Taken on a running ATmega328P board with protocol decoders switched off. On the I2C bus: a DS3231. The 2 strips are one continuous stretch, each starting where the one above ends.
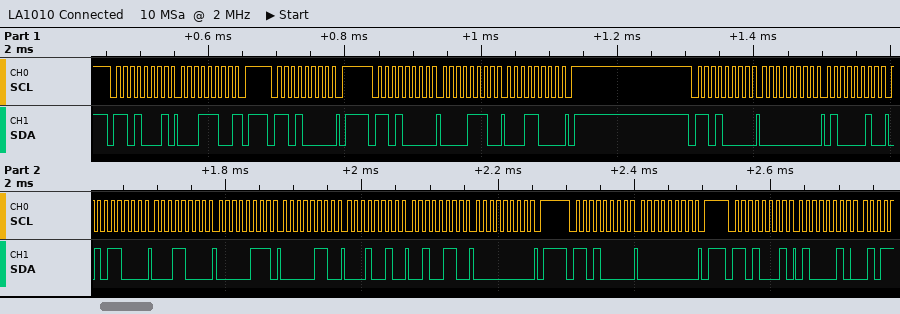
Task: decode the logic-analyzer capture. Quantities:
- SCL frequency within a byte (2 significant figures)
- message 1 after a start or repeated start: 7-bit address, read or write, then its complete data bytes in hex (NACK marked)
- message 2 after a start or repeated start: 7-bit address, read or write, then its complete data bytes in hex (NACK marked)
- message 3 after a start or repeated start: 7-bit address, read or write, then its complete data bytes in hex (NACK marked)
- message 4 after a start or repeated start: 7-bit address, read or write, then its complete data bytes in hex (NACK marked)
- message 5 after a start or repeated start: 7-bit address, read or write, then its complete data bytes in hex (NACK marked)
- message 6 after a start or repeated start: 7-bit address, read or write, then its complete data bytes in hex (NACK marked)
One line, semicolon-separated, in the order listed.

100 kHz; 0x68 read: 1C NACK; 0x68 write; 0x68 write: 0E 18; 0x68 write: 00 42 58 18 07 06 12 26 00; 0x68 write: 00; 0x68 read: 42
